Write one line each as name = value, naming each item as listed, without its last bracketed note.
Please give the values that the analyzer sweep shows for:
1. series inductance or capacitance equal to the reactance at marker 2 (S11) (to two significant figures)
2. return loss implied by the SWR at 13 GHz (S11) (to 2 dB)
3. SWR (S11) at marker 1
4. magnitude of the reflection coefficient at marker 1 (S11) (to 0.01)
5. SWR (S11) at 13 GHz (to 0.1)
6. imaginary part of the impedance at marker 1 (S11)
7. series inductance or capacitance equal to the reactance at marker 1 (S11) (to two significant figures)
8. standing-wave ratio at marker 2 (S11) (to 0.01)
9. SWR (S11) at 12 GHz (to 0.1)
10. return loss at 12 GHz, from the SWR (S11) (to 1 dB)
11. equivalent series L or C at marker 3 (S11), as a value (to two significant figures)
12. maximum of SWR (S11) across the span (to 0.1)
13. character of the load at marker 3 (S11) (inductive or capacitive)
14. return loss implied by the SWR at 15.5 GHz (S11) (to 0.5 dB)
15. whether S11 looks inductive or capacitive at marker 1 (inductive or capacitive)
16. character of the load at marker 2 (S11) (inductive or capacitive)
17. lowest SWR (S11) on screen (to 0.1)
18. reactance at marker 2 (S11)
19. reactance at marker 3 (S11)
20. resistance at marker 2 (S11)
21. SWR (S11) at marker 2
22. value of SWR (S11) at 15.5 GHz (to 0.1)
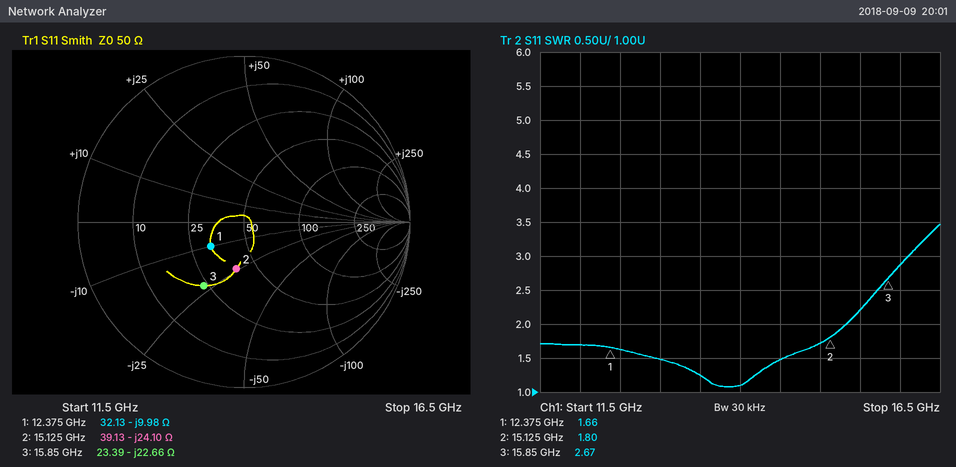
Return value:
series inductance or capacitance equal to the reactance at marker 2 (S11) = 440 fF
return loss implied by the SWR at 13 GHz (S11) = 14 dB
SWR (S11) at marker 1 = 1.66
magnitude of the reflection coefficient at marker 1 (S11) = 0.25
SWR (S11) at 13 GHz = 1.5
imaginary part of the impedance at marker 1 = -9.98 Ω
series inductance or capacitance equal to the reactance at marker 1 (S11) = 1.3 pF
standing-wave ratio at marker 2 (S11) = 1.80
SWR (S11) at 12 GHz = 1.7
return loss at 12 GHz, from the SWR (S11) = 12 dB
equivalent series L or C at marker 3 (S11), as a value = 440 fF
maximum of SWR (S11) across the span = 3.5
character of the load at marker 3 (S11) = capacitive
return loss implied by the SWR at 15.5 GHz (S11) = 8.5 dB
whether S11 looks inductive or capacitive at marker 1 = capacitive
character of the load at marker 2 (S11) = capacitive
lowest SWR (S11) on screen = 1.1
reactance at marker 2 = -24.10 Ω
reactance at marker 3 = -22.66 Ω
resistance at marker 2 = 39.13 Ω
SWR (S11) at marker 2 = 1.80
value of SWR (S11) at 15.5 GHz = 2.2
